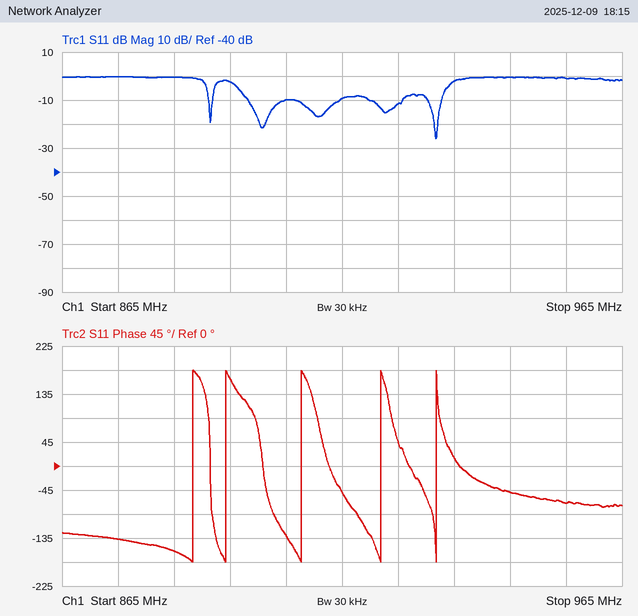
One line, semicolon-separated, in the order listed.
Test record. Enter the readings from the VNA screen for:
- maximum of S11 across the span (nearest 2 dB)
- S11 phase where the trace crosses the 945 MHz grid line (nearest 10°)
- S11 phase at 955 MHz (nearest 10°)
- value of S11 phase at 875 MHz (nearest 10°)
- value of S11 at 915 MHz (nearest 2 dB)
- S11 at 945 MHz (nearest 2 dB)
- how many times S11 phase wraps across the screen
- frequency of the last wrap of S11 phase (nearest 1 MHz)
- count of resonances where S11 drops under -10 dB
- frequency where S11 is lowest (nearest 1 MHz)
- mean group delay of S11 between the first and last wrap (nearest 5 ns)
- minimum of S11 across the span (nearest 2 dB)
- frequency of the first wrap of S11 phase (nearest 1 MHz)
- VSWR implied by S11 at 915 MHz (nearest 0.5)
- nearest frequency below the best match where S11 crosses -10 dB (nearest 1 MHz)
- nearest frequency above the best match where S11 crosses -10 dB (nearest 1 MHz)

0 dB; -50°; -70°; -140°; -10 dB; 0 dB; 5; 932 MHz; 5; 932 MHz; 90 ns; -26 dB; 888 MHz; 2.0; 930 MHz; 933 MHz
